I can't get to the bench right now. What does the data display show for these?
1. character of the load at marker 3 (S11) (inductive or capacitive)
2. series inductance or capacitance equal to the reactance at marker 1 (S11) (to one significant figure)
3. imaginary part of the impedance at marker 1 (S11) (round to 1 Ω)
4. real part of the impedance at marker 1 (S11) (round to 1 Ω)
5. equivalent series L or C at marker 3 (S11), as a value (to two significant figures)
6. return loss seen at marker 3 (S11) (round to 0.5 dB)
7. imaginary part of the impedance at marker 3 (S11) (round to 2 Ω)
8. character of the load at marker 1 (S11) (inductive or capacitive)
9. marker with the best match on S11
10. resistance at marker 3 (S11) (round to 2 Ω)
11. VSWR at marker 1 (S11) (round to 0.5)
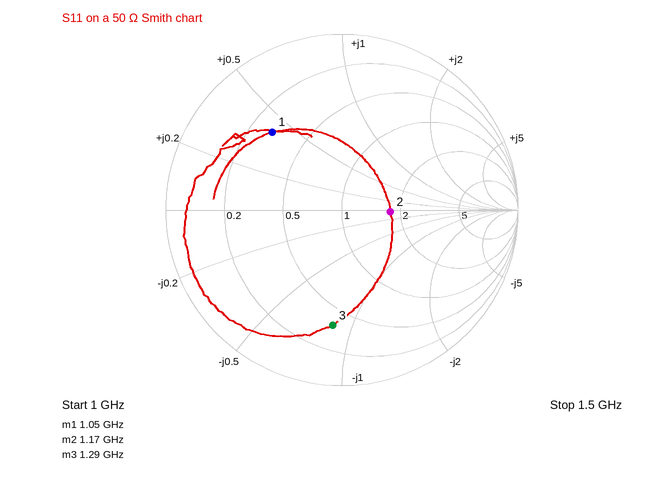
capacitive
3 nH
+21 Ω
15 Ω
2.9 pF
3.5 dB
-42 Ω
inductive
marker 2
18 Ω
4.0
